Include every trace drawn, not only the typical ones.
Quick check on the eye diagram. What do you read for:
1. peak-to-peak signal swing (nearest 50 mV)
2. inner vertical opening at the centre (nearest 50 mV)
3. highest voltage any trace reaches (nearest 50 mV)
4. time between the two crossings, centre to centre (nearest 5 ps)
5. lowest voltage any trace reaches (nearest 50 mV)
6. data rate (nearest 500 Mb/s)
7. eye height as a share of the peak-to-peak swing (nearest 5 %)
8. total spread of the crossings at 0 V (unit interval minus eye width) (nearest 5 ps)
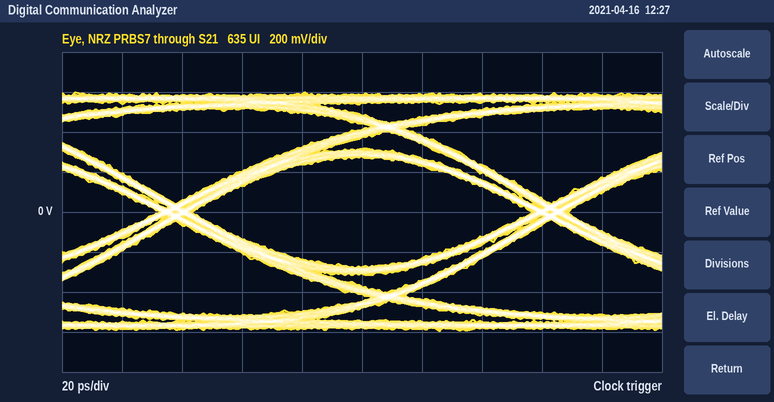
1.20 V
550 mV
600 mV
125 ps
-600 mV
8.0 Gb/s
45 %
10 ps
